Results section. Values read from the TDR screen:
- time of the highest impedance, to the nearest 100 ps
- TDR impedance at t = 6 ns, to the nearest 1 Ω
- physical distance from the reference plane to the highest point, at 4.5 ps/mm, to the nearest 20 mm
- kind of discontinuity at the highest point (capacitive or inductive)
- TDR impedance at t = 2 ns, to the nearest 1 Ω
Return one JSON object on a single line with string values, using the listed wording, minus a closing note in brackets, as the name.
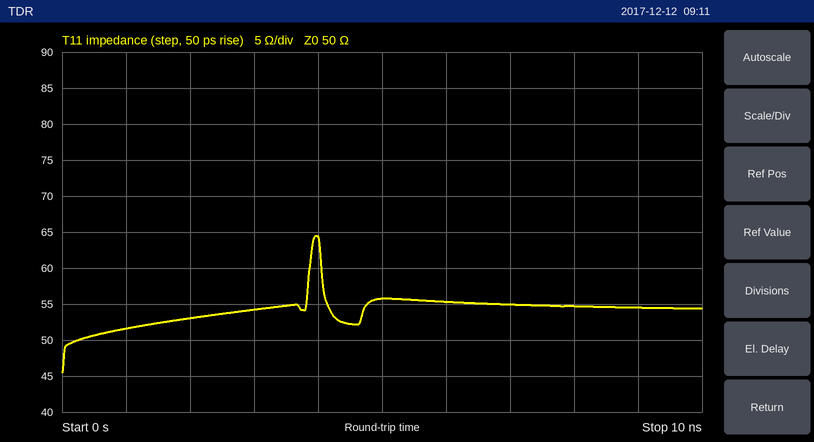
{"time of the highest impedance, to the nearest 100 ps": "4.0 ns", "TDR impedance at t = 6 ns, to the nearest 1 Ω": "55 Ω", "physical distance from the reference plane to the highest point, at 4.5 ps/mm, to the nearest 20 mm": "440 mm", "kind of discontinuity at the highest point": "inductive", "TDR impedance at t = 2 ns, to the nearest 1 Ω": "53 Ω"}
